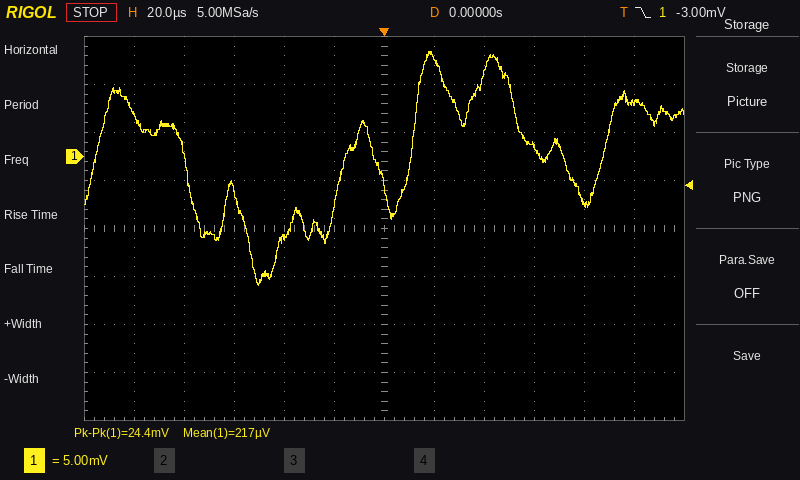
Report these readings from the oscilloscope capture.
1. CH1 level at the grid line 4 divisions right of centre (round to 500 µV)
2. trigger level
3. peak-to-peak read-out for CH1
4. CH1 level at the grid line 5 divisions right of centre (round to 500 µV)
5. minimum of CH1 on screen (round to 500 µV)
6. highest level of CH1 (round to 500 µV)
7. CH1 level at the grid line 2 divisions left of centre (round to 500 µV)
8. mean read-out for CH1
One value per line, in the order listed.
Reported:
-5.0 mV
-3.00 mV
24.4 mV
5.5 mV
-13.5 mV
11.0 mV
-8.5 mV
217 µV
